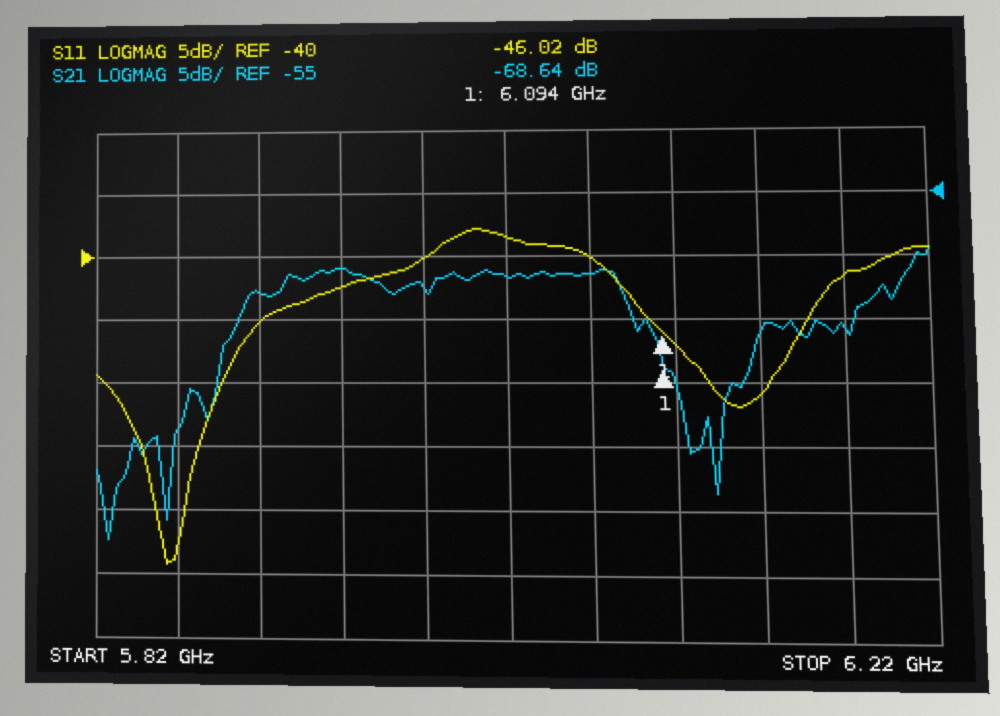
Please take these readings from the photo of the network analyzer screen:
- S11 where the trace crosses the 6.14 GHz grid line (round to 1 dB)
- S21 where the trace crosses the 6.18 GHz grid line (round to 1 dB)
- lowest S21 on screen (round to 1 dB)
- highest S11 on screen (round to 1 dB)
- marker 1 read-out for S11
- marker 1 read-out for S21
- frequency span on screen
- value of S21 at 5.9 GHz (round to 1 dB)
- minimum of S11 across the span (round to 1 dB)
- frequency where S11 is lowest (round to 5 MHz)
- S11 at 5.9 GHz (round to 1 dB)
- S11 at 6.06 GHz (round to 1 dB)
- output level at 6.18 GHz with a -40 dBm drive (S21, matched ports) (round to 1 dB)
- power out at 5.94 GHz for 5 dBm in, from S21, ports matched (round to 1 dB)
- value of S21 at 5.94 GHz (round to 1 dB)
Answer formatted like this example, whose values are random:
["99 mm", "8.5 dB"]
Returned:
["-51 dB", "-66 dB", "-82 dB", "-38 dB", "-46.02 dB", "-68.64 dB", "400 MHz", "-63 dB", "-64 dB", "5.855 GHz", "-45 dB", "-40 dB", "-106 dBm", "-56 dBm", "-61 dB"]
